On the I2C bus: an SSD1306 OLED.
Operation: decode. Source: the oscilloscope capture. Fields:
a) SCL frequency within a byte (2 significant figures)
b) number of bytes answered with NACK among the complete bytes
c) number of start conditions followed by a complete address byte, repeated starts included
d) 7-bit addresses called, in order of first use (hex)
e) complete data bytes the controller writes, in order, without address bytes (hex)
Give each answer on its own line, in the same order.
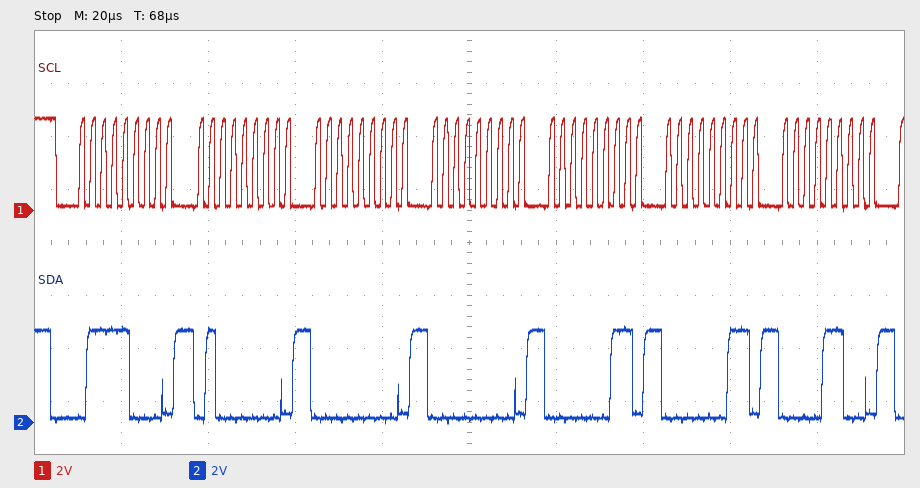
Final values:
400 kHz
0
1
0x3C
40 00 00 03 03 0C
